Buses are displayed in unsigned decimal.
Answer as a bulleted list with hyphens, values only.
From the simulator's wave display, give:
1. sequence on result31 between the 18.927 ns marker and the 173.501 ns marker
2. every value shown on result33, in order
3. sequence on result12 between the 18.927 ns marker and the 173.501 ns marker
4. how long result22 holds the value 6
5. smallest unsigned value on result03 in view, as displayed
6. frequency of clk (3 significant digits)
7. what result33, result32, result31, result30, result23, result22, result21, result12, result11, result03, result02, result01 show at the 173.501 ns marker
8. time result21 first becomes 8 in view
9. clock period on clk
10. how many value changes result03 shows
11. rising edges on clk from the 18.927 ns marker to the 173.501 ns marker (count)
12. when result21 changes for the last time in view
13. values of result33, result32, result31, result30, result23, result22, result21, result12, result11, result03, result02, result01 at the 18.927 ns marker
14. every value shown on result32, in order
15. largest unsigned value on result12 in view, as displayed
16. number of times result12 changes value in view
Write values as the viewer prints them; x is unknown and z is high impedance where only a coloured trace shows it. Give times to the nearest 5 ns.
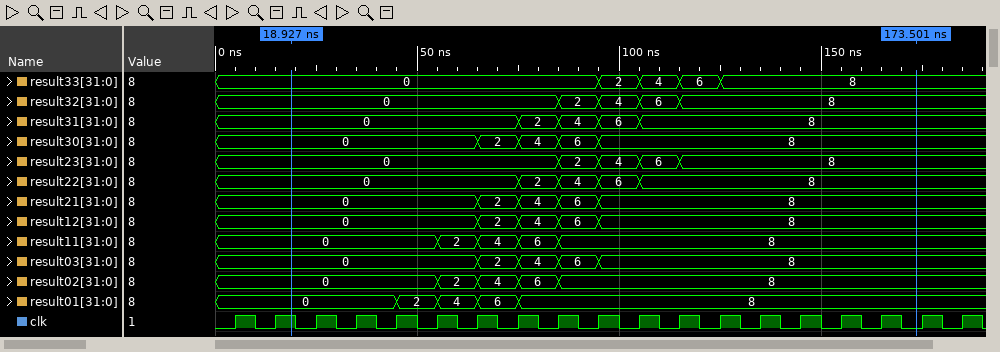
- 0, 2, 4, 6, 8
- 0, 2, 4, 6, 8
- 0, 2, 4, 6, 8
- 10 ns
- 0
- 100 MHz
- result33=8, result32=8, result31=8, result30=8, result23=8, result22=8, result21=8, result12=8, result11=8, result03=8, result02=8, result01=8
- 95 ns
- 10 ns
- 4
- 15
- 95 ns
- result33=0, result32=0, result31=0, result30=0, result23=0, result22=0, result21=0, result12=0, result11=0, result03=0, result02=0, result01=0
- 0, 2, 4, 6, 8
- 8
- 4
